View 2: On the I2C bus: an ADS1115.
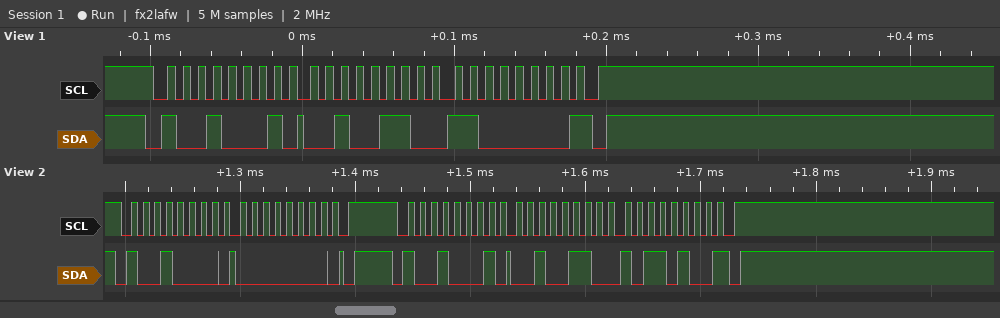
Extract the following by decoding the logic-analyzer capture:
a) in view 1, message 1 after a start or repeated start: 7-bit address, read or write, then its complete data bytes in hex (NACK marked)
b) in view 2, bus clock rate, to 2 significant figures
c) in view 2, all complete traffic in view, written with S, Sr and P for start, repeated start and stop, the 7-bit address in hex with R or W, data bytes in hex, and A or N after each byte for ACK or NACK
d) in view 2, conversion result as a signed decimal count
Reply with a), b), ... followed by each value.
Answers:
a) 0x48 read: 26 C0 NACK
b) 100 kHz
c) S 48W A 00 A P S 48R A 26 A B4 N P
d) 9908
